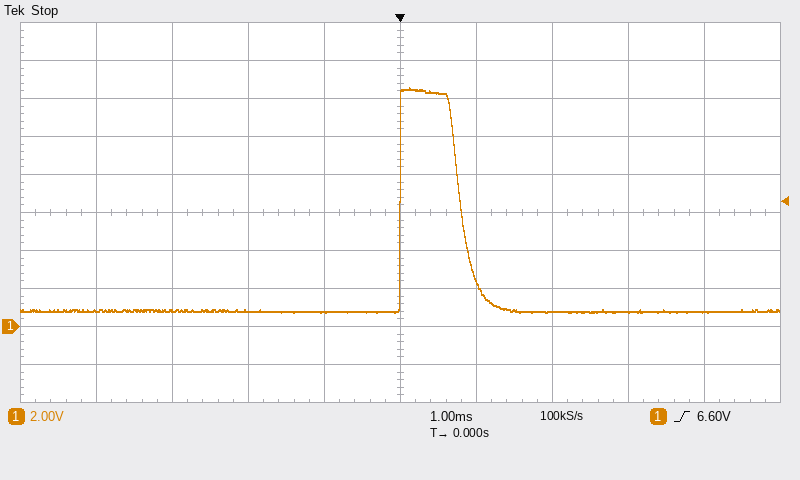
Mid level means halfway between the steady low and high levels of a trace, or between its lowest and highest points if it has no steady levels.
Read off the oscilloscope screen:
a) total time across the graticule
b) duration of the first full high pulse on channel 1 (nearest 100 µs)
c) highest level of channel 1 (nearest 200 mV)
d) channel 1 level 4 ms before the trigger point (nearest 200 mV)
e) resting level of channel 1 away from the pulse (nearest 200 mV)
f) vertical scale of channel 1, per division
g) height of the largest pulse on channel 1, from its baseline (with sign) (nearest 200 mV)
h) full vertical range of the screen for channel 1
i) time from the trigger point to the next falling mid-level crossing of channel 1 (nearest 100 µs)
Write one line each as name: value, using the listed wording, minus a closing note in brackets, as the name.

total time across the graticule: 10 ms
duration of the first full high pulse on channel 1: 800 µs
highest level of channel 1: 12.6 V
channel 1 level 4 ms before the trigger point: 800 mV
resting level of channel 1 away from the pulse: 800 mV
vertical scale of channel 1, per division: 2 V
height of the largest pulse on channel 1, from its baseline (with sign): +11.8 V
full vertical range of the screen for channel 1: 20 V
time from the trigger point to the next falling mid-level crossing of channel 1: 800 µs
